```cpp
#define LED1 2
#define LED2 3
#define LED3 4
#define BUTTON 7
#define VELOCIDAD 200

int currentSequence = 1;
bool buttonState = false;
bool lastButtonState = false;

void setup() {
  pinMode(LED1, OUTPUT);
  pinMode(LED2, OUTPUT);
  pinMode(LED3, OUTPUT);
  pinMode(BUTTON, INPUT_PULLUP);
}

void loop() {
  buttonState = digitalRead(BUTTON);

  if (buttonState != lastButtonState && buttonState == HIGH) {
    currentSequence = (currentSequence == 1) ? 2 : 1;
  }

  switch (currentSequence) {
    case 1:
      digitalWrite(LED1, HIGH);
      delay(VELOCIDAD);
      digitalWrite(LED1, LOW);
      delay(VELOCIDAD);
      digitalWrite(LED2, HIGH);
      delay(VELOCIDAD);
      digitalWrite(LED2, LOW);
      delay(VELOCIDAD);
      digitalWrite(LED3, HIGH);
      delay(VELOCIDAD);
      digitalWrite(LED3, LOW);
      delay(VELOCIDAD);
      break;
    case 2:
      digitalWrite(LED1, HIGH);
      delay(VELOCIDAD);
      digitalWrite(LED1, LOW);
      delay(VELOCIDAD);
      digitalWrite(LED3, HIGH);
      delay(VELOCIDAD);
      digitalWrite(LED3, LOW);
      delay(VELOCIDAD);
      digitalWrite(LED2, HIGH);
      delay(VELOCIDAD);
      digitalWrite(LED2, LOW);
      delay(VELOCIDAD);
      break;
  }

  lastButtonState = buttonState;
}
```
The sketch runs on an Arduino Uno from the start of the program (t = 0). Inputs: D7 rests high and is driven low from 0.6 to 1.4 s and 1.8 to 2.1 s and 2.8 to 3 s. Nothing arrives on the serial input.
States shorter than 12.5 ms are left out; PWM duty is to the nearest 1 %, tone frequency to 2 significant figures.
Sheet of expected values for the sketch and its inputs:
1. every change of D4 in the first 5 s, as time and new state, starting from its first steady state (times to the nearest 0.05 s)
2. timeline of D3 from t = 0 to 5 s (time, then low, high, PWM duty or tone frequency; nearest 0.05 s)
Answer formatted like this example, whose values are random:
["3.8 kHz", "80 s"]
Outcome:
["0 s low; 0.4 s high; 0.6 s low; 1.6 s high; 1.8 s low; 3.2 s high; 3.4 s low; 4.4 s high; 4.6 s low", "0 s low; 0.8 s high; 1 s low; 2 s high; 2.2 s low; 2.8 s high; 3 s low; 4 s high; 4.2 s low"]
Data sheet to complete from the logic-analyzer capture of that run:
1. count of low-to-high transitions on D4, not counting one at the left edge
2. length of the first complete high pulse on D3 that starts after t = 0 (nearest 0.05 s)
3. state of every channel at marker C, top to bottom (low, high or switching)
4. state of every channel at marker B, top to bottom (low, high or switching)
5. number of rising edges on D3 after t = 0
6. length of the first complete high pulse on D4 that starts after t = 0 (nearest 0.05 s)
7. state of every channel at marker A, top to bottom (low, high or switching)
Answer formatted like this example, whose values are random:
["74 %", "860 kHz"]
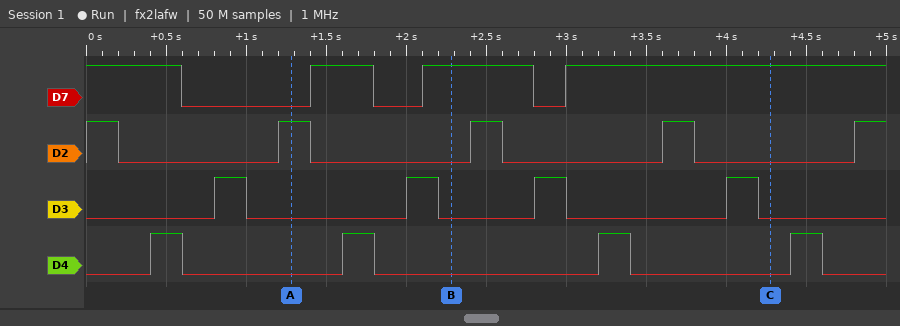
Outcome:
["4", "0.20 s", "D7 high, D2 low, D3 low, D4 low", "D7 high, D2 low, D3 low, D4 low", "4", "0.20 s", "D7 low, D2 high, D3 low, D4 low"]
